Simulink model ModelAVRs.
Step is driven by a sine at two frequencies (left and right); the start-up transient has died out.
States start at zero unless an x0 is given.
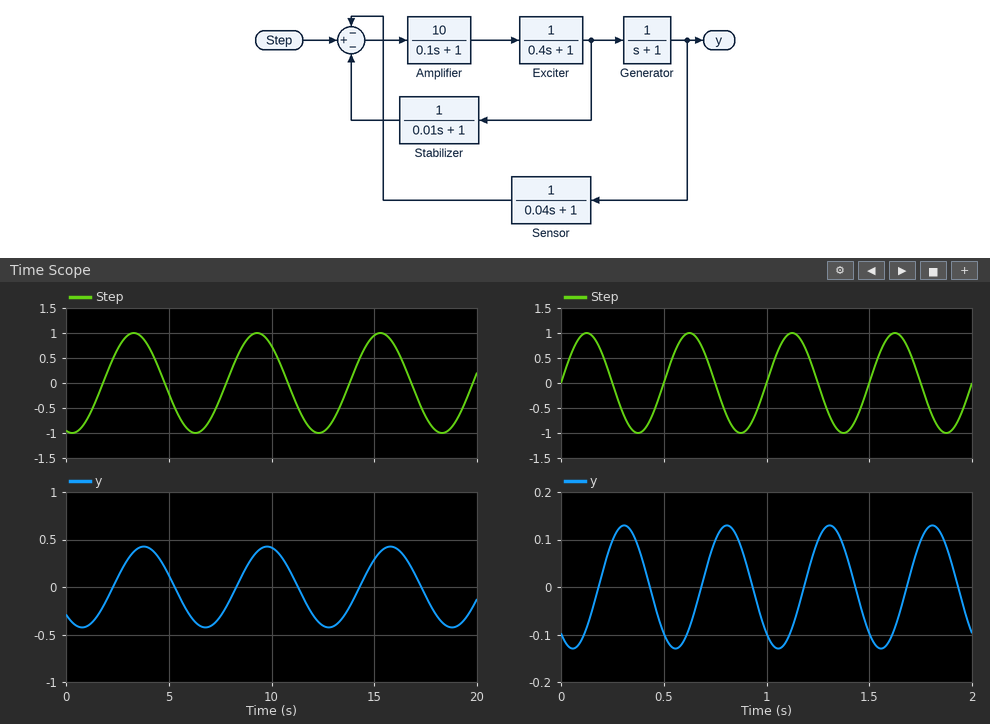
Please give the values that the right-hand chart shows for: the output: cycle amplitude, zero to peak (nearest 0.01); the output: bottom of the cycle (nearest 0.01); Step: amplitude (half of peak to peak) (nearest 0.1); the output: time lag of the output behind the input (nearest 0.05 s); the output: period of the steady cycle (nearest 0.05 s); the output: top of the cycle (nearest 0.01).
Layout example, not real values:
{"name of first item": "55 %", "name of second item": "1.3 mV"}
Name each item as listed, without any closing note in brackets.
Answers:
{"the output: cycle amplitude, zero to peak": "0.13", "the output: bottom of the cycle": "-0.13", "Step: amplitude (half of peak to peak)": "1.0", "the output: time lag of the output behind the input": "0.20 s", "the output: period of the steady cycle": "0.50 s", "the output: top of the cycle": "0.13"}
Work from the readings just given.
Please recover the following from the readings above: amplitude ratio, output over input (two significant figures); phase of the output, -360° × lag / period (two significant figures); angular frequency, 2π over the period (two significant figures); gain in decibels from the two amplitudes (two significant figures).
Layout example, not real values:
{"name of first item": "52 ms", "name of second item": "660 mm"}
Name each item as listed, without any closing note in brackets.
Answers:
{"amplitude ratio, output over input": "0.13", "phase of the output, -360° × lag / period": "-140°", "angular frequency, 2π over the period": "13 rad/s", "gain in decibels from the two amplitudes": "-18 dB"}
